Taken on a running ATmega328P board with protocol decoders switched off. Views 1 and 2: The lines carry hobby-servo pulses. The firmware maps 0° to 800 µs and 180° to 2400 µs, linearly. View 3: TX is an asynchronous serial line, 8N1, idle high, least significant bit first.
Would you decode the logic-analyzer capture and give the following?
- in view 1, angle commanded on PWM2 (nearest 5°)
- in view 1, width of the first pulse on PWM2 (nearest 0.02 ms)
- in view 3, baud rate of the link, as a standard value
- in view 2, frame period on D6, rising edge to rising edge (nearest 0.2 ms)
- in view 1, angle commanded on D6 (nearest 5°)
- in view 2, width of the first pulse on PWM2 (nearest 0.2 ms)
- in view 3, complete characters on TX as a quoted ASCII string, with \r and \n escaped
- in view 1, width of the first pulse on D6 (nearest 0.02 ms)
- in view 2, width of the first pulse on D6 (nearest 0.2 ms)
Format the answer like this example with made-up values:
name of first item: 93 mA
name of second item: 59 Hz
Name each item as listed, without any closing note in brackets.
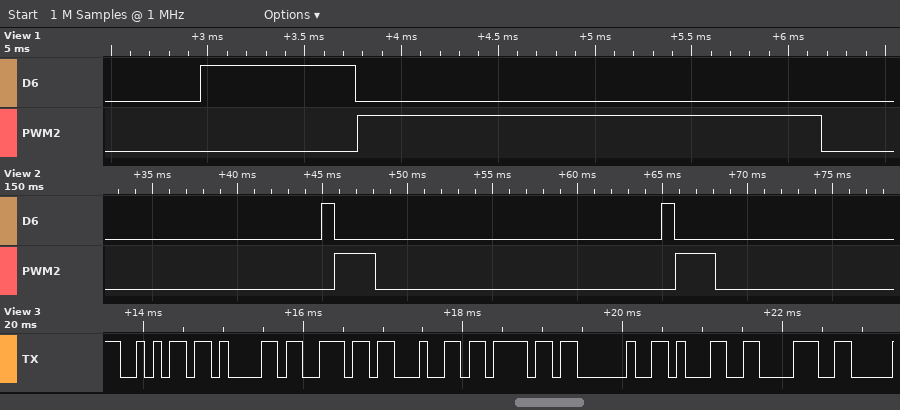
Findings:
in view 1, angle commanded on PWM2: 180°
in view 1, width of the first pulse on PWM2: 2.40 ms
in view 3, baud rate of the link, as a standard value: 9600 baud
in view 2, frame period on D6, rising edge to rising edge: 20.0 ms
in view 1, angle commanded on D6: 0°
in view 2, width of the first pulse on PWM2: 2.4 ms
in view 3, complete characters on TX as a quoted ASCII string, with \r and \n escaped: "jando 18"
in view 1, width of the first pulse on D6: 0.80 ms
in view 2, width of the first pulse on D6: 0.8 ms
